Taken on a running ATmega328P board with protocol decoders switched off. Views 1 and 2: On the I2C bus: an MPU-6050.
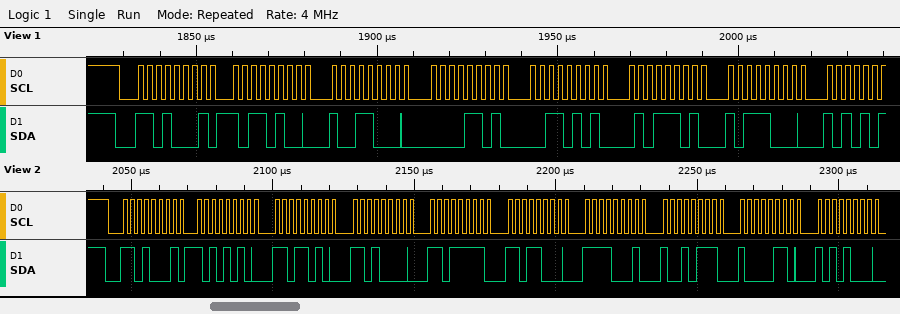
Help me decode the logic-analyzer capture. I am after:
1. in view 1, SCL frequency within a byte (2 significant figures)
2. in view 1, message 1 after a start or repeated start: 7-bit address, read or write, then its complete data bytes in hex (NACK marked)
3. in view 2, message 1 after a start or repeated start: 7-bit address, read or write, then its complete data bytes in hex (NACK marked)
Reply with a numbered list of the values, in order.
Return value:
1. 400 kHz
2. 0x68 read: B4 98 0D 35 5D B8
3. 0x68 read: AA DA D0 DF D8 F1 97 86 A8
